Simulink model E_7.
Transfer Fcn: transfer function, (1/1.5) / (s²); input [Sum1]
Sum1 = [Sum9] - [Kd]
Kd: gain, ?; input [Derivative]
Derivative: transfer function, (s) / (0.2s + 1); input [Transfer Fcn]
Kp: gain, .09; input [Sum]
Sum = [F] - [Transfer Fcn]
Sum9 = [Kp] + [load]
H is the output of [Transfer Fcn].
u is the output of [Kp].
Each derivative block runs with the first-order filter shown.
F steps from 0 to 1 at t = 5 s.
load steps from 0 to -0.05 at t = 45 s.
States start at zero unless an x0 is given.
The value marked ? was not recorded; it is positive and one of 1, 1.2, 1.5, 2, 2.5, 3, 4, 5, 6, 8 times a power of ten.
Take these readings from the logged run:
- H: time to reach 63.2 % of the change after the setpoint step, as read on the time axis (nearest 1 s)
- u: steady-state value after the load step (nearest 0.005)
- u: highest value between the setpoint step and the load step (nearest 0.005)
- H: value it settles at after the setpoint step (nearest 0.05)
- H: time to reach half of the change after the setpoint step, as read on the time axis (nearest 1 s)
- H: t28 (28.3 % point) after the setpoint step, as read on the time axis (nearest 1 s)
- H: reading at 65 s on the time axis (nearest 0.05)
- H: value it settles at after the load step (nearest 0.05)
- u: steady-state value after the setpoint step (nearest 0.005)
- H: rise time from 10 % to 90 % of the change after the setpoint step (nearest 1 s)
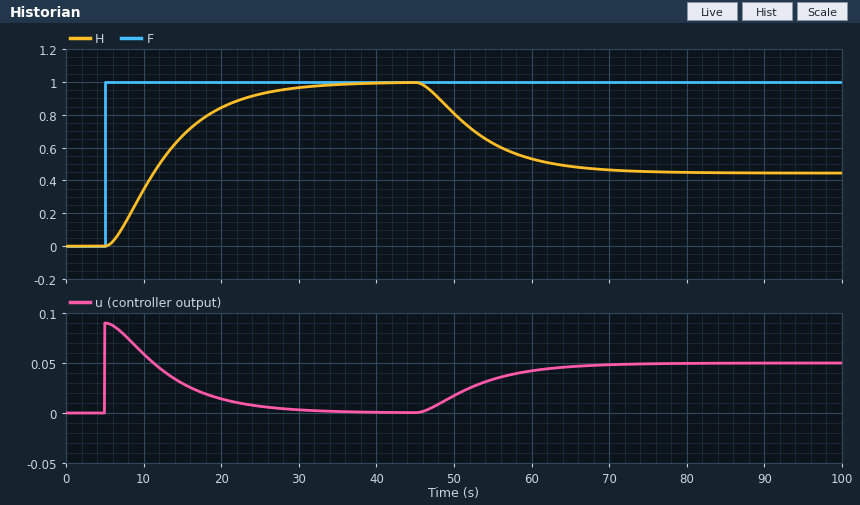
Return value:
14 s
0.050
0.090
1.00
12 s
9 s
0.50
0.45
0.000
16 s
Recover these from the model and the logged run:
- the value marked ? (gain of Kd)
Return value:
0.8
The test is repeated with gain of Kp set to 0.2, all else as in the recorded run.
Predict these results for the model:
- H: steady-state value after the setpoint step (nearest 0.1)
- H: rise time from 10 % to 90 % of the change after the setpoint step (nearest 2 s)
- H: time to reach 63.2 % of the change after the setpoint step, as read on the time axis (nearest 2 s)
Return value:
1.0
6 s
10 s
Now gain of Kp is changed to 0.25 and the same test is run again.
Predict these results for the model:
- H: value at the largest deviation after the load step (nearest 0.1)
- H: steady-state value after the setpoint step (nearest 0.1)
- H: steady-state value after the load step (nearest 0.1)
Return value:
0.8
1.0
0.8
